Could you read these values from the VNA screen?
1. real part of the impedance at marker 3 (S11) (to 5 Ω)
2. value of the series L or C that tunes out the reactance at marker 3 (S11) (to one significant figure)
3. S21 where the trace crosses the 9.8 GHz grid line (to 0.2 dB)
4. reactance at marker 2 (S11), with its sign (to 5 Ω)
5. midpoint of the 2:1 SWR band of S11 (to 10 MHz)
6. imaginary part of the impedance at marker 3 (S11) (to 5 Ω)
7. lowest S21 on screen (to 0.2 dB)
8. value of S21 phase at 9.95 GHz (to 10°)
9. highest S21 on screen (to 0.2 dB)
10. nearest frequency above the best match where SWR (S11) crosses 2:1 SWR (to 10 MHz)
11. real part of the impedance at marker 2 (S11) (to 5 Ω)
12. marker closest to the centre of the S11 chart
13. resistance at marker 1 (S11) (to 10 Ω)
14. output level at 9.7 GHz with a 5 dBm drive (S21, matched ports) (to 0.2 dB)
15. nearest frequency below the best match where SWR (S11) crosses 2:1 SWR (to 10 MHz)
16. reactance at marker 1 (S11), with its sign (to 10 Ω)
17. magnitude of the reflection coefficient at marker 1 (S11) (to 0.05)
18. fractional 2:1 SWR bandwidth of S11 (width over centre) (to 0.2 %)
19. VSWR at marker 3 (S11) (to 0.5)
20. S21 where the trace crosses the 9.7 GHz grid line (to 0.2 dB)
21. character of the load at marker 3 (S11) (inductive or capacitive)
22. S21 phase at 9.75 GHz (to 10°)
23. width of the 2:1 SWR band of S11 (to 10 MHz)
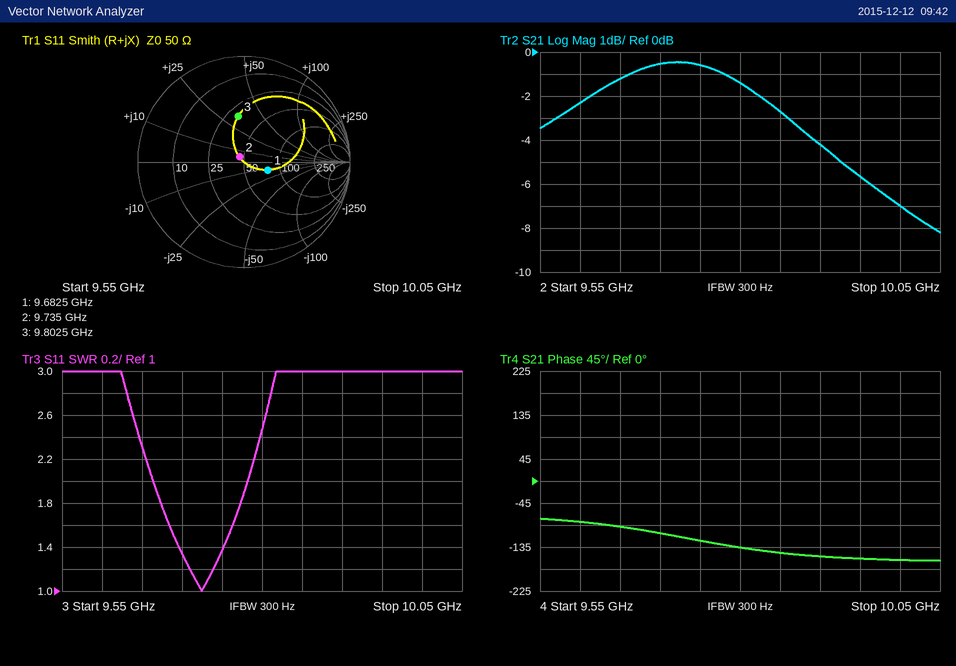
30 Ω
500 fF
-1.4 dB
+5 Ω
9.72 GHz
+35 Ω
-8.2 dB
-160°
-0.4 dB
9.78 GHz
45 Ω
marker 2
80 Ω
4.4 dBm
9.66 GHz
-10 Ω
0.25
1.2 %
2.5
-0.6 dB
inductive
-120°
120 MHz
